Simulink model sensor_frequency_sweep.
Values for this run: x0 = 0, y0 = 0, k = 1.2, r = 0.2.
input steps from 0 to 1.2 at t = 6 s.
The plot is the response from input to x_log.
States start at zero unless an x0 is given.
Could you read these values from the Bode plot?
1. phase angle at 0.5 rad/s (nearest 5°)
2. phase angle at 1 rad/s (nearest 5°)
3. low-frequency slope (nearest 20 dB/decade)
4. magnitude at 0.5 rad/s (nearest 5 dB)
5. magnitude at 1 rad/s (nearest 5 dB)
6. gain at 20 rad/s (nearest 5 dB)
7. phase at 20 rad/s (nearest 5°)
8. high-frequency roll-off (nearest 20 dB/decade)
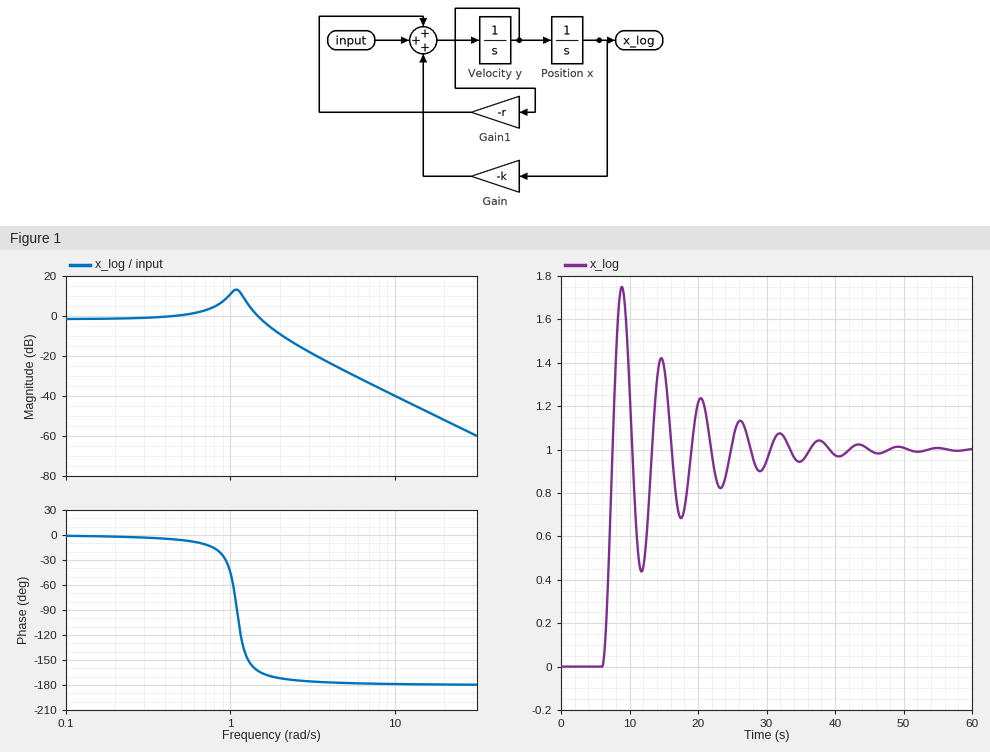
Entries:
-5°
-45°
0 dB/decade
0 dB
10 dB
-50 dB
-180°
-40 dB/decade
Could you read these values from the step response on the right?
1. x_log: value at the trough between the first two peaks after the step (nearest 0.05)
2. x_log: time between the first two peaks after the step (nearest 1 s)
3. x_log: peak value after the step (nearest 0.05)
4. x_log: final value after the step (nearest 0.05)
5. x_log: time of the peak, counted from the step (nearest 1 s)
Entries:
0.45
6 s
1.75
1.00
3 s
